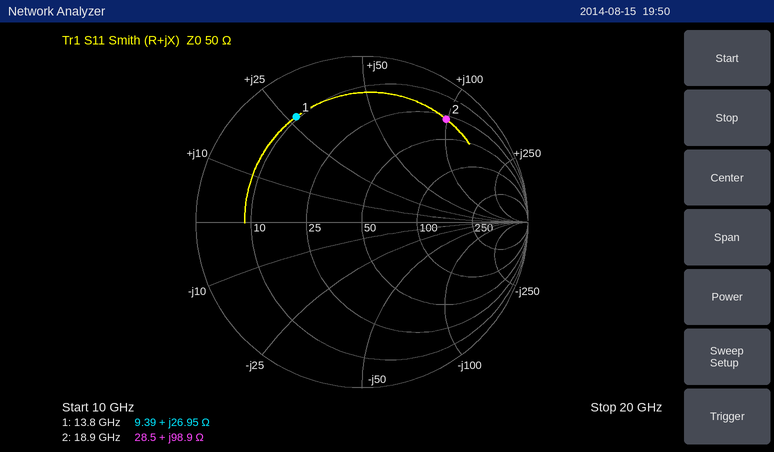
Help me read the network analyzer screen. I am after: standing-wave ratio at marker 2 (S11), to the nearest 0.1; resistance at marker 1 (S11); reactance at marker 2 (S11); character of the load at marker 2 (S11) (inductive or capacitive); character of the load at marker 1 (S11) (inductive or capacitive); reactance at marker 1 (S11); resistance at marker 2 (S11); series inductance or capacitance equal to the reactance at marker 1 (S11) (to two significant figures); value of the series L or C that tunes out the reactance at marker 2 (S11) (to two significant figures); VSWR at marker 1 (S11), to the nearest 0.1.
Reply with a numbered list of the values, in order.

1. 9.1
2. 9.39 Ω
3. +98.9 Ω
4. inductive
5. inductive
6. +26.95 Ω
7. 28.5 Ω
8. 310 pH
9. 85 fF
10. 6.9
